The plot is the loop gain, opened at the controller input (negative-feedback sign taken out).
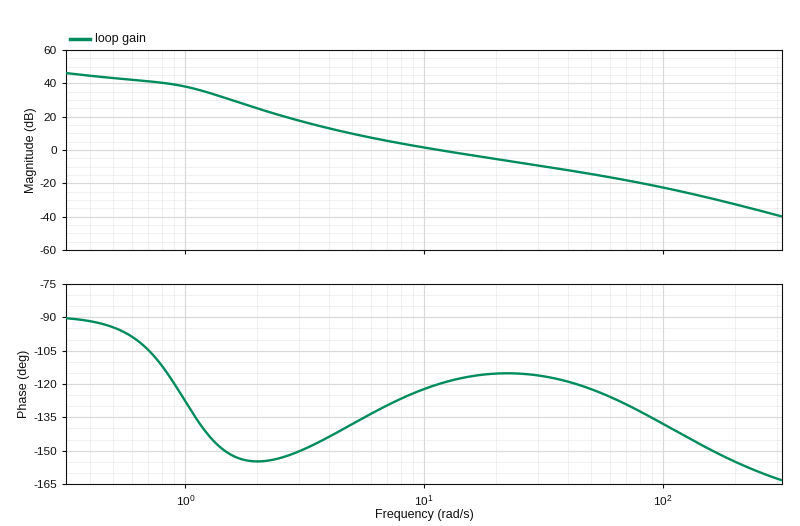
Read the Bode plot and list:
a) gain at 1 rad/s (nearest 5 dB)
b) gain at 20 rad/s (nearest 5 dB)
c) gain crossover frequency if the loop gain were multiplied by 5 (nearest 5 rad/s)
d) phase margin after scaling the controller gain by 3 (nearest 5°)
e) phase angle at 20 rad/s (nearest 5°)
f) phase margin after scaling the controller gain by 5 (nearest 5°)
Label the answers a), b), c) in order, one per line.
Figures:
a) 40 dB
b) -5 dB
c) 50 rad/s
d) 65°
e) -115°
f) 60°
